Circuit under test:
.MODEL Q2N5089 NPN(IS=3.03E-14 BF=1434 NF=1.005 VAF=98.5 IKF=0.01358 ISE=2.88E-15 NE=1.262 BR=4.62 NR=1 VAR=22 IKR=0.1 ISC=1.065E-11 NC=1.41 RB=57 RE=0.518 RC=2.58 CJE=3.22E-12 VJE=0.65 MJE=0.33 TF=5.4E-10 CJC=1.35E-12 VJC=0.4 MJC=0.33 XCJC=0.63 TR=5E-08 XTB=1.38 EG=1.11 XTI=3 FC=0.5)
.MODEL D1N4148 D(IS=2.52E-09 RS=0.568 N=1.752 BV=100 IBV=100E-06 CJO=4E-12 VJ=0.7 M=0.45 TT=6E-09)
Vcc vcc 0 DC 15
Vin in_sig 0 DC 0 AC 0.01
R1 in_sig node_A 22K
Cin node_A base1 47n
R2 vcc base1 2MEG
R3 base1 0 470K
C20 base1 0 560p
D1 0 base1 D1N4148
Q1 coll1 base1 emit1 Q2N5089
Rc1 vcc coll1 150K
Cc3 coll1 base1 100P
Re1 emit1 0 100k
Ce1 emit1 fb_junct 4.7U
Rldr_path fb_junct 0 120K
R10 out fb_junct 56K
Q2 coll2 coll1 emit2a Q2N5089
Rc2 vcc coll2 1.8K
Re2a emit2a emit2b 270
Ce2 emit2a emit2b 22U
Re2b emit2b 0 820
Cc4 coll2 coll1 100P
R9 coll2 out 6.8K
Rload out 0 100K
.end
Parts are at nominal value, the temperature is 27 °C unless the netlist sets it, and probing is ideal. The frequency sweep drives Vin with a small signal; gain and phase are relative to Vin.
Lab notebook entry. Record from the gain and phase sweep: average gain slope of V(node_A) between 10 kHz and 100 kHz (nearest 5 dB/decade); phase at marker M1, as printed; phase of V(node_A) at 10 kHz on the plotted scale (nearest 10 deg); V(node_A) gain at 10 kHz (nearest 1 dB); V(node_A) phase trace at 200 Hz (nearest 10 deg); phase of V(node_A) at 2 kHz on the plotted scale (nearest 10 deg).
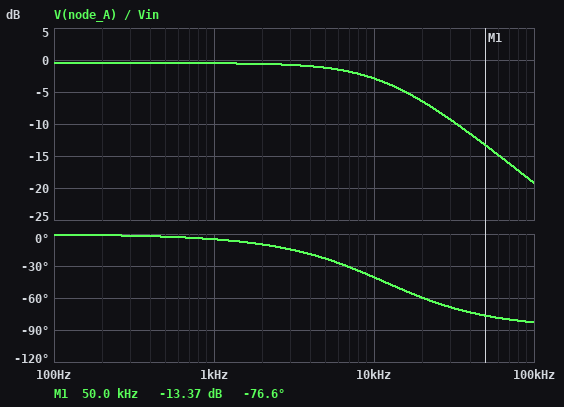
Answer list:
-15 dB/decade
-76.6 deg
-40 deg
-3 dB
0 deg
-10 deg
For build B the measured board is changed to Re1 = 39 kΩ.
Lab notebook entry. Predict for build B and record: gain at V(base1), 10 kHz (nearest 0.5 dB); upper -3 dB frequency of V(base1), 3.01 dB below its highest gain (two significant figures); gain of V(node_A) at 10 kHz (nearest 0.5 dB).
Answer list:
-4.0 dB
9.5 kHz
-3.5 dB
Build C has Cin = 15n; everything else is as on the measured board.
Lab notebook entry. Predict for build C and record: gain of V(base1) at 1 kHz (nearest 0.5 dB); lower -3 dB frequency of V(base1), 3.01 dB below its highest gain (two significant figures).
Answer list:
-1.0 dB
26 Hz
